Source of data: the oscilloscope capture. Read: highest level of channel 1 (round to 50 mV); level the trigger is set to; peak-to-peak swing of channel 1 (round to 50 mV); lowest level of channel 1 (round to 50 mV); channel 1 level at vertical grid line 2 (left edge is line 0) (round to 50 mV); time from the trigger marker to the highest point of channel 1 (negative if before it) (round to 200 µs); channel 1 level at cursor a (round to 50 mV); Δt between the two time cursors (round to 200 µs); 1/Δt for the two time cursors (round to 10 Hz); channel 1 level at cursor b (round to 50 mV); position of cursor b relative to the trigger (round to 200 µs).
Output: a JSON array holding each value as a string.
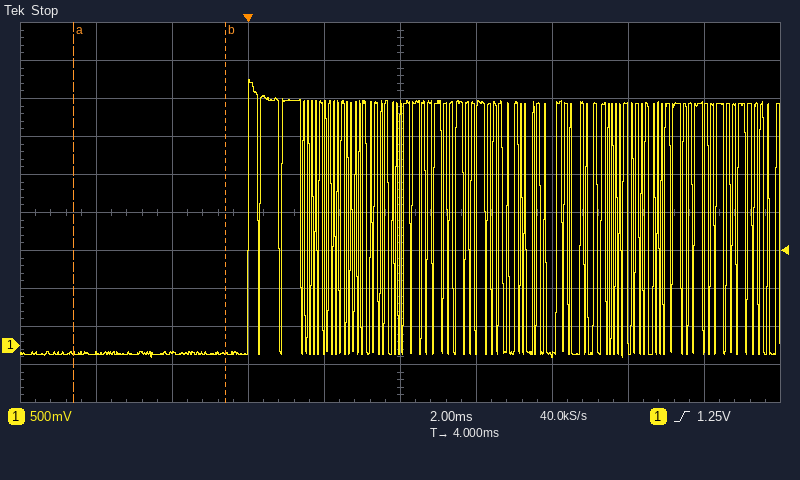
["3.50 V", "1.25 V", "3.65 V", "-150 mV", "-100 mV", "0.0 ms", "-100 mV", "4.0 ms", "250 Hz", "-100 mV", "-600 µs"]
